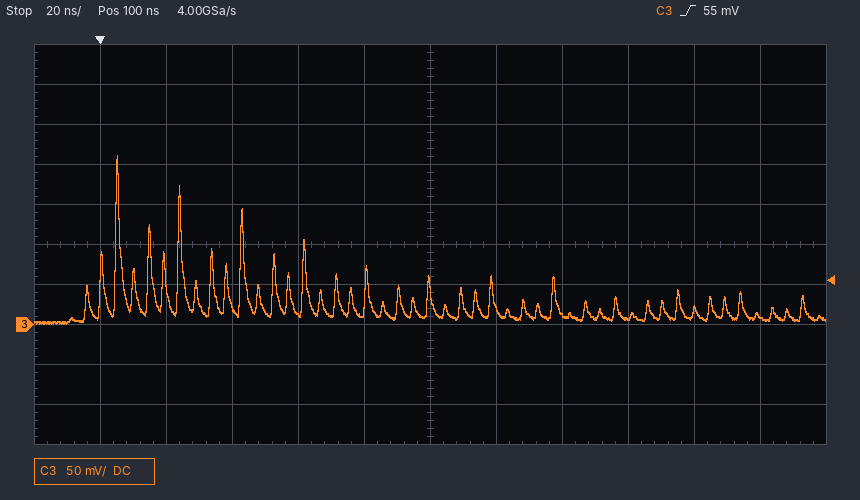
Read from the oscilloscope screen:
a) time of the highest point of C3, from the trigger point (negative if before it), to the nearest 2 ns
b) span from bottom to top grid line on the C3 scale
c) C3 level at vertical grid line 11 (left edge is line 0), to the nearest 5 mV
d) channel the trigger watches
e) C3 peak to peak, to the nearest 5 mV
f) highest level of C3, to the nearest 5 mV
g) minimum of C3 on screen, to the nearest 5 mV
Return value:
+6 ns
500 mV
10 mV
C3
210 mV
210 mV
0 mV
